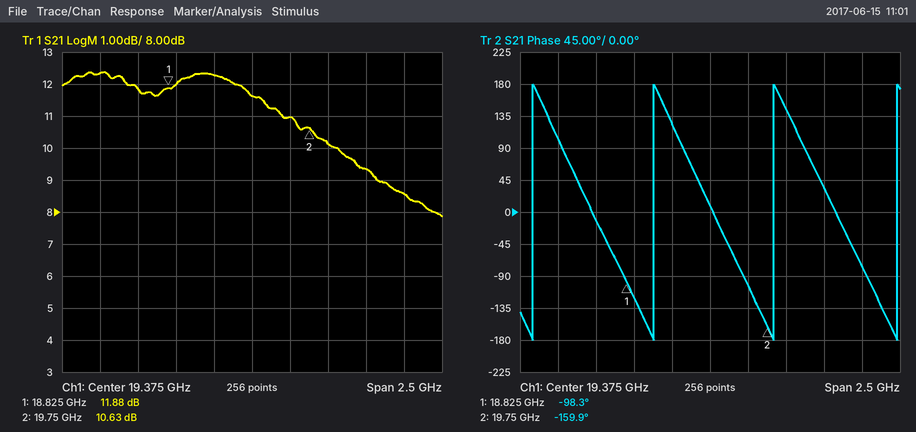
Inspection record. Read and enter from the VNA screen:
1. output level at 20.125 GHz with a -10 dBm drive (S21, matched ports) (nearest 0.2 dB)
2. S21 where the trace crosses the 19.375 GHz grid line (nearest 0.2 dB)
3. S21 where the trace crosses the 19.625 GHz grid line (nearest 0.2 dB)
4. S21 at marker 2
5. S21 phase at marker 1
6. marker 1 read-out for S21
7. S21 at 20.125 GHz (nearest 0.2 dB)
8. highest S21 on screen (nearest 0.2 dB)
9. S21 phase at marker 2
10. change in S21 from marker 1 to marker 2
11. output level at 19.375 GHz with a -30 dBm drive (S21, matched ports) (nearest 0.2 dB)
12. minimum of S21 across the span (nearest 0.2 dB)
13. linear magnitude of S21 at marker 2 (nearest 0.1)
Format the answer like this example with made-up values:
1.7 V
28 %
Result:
-0.6 dBm
11.6 dB
11.0 dB
10.63 dB
-98.3°
11.88 dB
9.4 dB
12.4 dB
-159.9°
-1.25 dB
-18.4 dBm
7.8 dB
3.4
